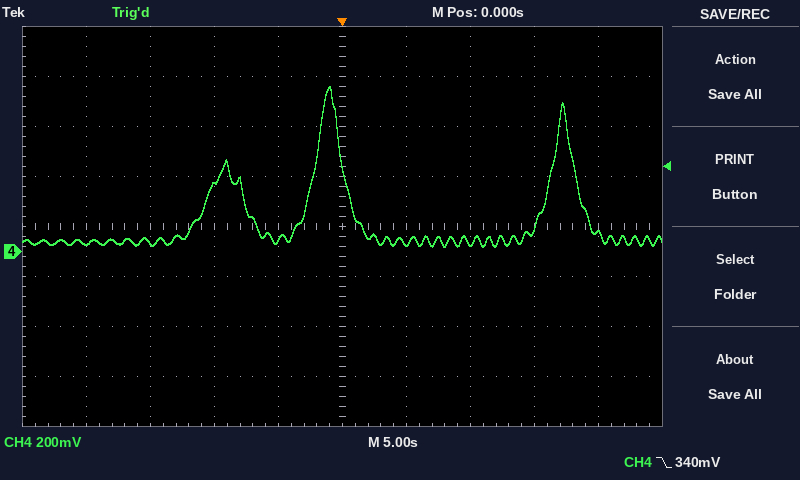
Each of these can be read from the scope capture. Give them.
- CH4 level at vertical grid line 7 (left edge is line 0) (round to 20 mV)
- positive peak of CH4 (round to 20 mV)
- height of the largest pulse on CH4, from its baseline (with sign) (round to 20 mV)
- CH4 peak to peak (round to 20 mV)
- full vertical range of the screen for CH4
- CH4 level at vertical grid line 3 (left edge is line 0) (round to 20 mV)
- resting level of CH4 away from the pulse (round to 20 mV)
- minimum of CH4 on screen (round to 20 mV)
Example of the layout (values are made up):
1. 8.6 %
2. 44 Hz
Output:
1. 40 mV
2. 660 mV
3. +620 mV
4. 640 mV
5. 1.6 V
6. 260 mV
7. 40 mV
8. 20 mV
